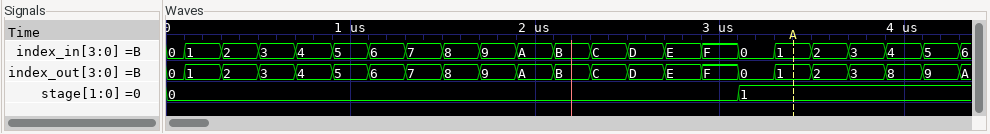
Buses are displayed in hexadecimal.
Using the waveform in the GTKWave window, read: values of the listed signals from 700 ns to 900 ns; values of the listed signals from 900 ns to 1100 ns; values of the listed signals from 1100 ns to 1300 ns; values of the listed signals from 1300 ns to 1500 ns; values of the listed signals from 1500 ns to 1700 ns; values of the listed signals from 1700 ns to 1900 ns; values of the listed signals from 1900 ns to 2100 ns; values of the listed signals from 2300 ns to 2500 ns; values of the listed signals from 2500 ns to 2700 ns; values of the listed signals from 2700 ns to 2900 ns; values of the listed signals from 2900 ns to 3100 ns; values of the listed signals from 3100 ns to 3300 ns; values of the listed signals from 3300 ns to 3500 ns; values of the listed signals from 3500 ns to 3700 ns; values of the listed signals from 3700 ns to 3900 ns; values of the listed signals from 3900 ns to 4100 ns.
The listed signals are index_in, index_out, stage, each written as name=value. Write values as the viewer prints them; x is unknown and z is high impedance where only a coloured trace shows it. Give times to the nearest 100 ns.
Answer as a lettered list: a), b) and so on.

a) index_in=4, index_out=4, stage=0
b) index_in=5, index_out=5, stage=0
c) index_in=6, index_out=6, stage=0
d) index_in=7, index_out=7, stage=0
e) index_in=8, index_out=8, stage=0
f) index_in=9, index_out=9, stage=0
g) index_in=A, index_out=A, stage=0
h) index_in=C, index_out=C, stage=0
i) index_in=D, index_out=D, stage=0
j) index_in=E, index_out=E, stage=0
k) index_in=F, index_out=F, stage=0
l) index_in=0, index_out=0, stage=1
m) index_in=1, index_out=1, stage=1
n) index_in=2, index_out=2, stage=1
o) index_in=3, index_out=3, stage=1
p) index_in=4, index_out=8, stage=1
